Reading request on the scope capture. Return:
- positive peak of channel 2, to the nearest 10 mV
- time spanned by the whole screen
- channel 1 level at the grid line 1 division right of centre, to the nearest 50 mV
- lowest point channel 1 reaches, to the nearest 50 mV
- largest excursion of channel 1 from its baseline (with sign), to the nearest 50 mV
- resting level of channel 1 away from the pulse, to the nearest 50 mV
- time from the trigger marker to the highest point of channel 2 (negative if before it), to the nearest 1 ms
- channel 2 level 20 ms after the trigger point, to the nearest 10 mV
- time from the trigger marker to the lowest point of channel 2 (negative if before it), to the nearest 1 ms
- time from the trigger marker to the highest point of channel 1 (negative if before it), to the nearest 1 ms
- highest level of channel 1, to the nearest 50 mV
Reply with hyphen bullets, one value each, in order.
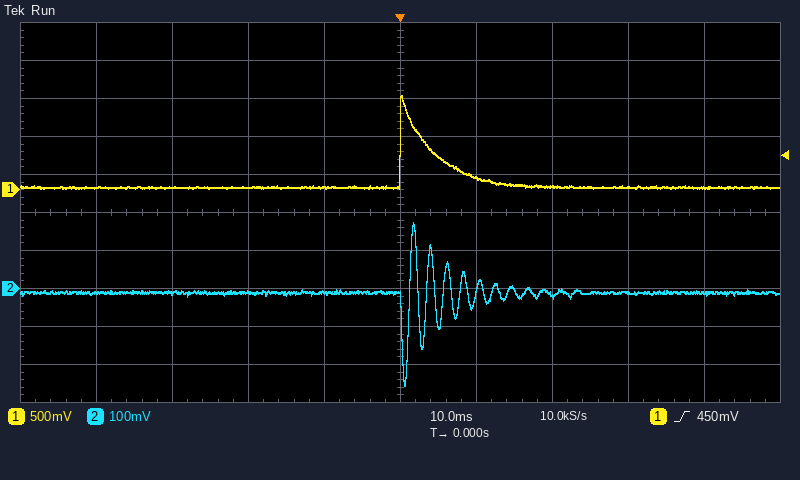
- 170 mV
- 100 ms
- 150 mV
- 0 mV
- +1.20 V
- 50 mV
- +2 ms
- -20 mV
- +1 ms
- 0 ms
- 1.25 V
